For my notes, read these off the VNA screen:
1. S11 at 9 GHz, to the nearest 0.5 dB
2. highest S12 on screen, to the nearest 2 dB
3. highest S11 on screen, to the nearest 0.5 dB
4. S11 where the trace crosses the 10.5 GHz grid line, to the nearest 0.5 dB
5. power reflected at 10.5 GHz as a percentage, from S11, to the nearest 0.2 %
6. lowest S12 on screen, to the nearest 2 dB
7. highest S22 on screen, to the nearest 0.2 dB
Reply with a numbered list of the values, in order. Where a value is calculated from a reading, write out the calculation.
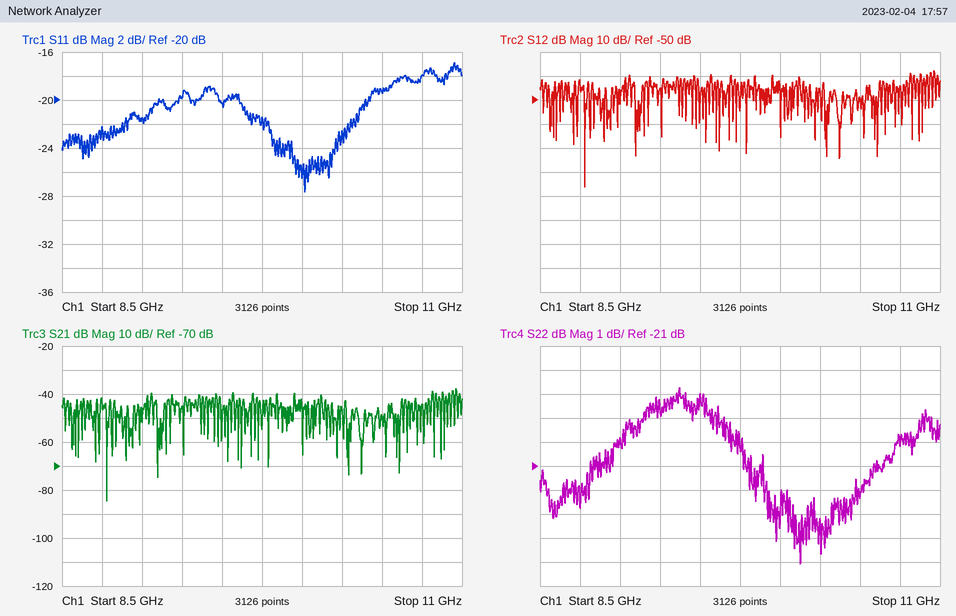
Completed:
1. -21.5 dB
2. -38 dB
3. -17.0 dB
4. -19.5 dB
5. 10^(-19.5/10) ≈ 1.12 %, so 1.2 % to the nearest 0.2 %
6. -86 dB
7. -17.8 dB
